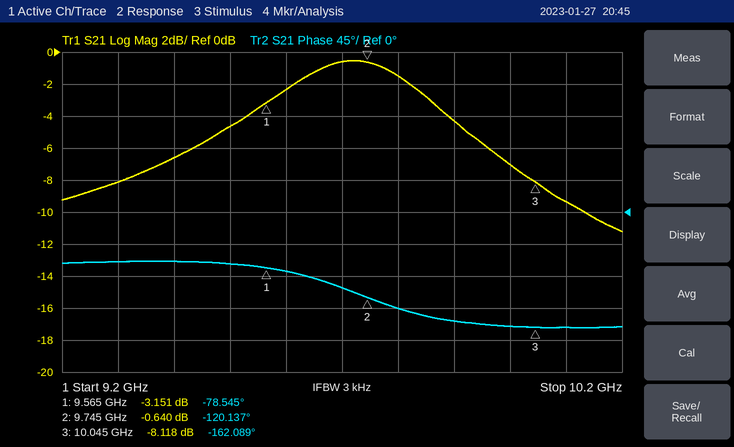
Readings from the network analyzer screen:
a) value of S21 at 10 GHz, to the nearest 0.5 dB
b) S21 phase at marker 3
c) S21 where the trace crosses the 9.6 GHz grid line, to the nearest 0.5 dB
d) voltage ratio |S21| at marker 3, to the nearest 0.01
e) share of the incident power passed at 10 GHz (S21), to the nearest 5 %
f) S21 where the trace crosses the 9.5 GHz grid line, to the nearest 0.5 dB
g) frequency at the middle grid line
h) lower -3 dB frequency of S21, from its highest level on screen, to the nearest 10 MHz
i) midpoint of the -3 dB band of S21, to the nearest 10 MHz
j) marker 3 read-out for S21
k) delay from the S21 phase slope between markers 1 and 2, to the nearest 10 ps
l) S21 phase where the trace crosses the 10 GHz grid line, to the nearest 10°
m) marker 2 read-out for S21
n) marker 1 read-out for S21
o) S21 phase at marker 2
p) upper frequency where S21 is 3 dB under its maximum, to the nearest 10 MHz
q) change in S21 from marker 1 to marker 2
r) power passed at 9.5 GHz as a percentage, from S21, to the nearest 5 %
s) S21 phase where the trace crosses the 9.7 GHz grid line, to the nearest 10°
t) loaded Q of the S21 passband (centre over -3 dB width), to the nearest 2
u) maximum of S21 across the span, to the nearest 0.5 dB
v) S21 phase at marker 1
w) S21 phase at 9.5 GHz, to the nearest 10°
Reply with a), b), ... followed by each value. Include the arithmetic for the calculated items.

a) -7.0 dB
b) -162.089°
c) -2.5 dB
d) 10^(-8.118/20) ≈ 0.39
e) 10^(-7/10) ≈ 20 %
f) -4.5 dB
g) 9.7 GHz
h) 9.55 GHz
i) 9.71 GHz
j) -8.118 dB
k) −(-120.137° − (-78.545°))/(360° × 180 MHz) ≈ 642 ps, so 640 ps to the nearest 10 ps
l) -160°
m) -0.640 dB
n) -3.151 dB
o) -120.137°
p) 9.87 GHz
q) -0.64 − (-3.151) = 2.511 dB
r) 10^(-4.5/10) ≈ 35 %
s) -110°
t) 9.71 GHz / 320 MHz ≈ 30
u) -0.5 dB
v) -78.545°
w) -70°
